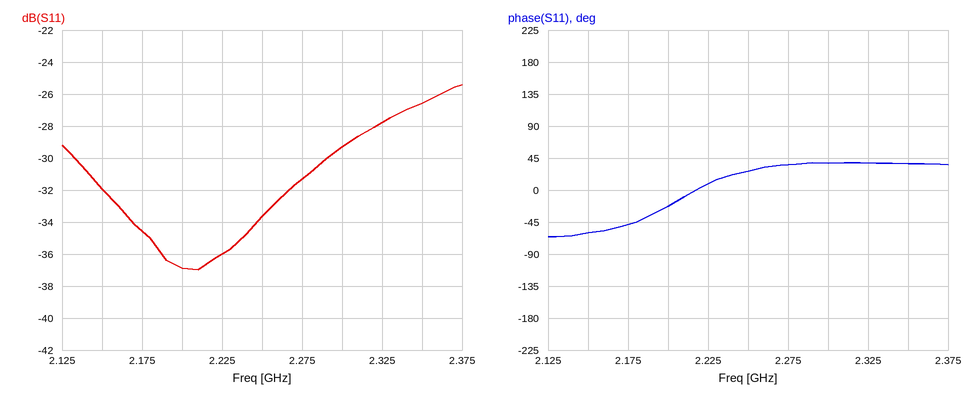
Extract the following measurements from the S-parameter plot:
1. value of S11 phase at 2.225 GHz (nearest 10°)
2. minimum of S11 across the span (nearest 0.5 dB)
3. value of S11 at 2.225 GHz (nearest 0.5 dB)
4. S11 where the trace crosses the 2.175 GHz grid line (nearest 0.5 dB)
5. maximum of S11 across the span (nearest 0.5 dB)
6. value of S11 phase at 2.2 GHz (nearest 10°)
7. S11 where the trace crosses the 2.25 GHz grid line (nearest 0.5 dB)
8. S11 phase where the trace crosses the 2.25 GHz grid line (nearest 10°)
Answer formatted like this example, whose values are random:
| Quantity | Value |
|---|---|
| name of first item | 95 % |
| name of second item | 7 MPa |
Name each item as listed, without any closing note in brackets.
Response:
| Quantity | Value |
|---|---|
| value of S11 phase at 2.225 GHz | 10° |
| minimum of S11 across the span | -37.0 dB |
| value of S11 at 2.225 GHz | -36.0 dB |
| S11 where the trace crosses the 2.175 GHz grid line | -34.5 dB |
| maximum of S11 across the span | -25.5 dB |
| value of S11 phase at 2.2 GHz | -20° |
| S11 where the trace crosses the 2.25 GHz grid line | -33.5 dB |
| S11 phase where the trace crosses the 2.25 GHz grid line | 30° |
